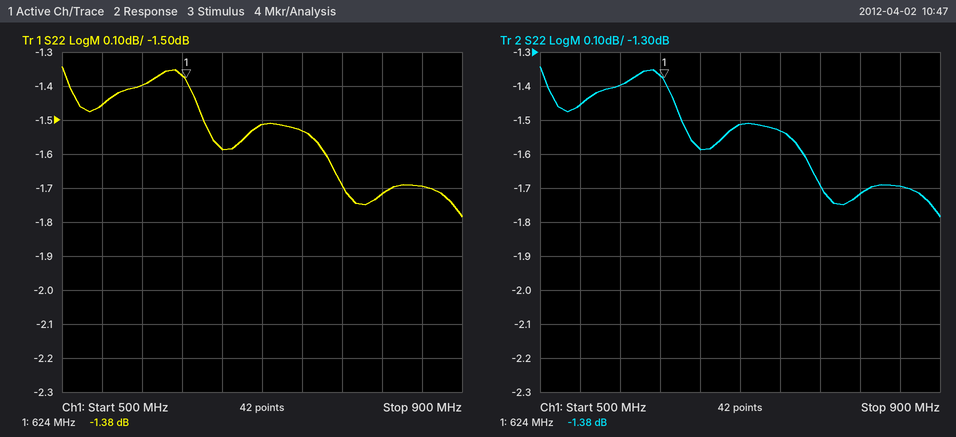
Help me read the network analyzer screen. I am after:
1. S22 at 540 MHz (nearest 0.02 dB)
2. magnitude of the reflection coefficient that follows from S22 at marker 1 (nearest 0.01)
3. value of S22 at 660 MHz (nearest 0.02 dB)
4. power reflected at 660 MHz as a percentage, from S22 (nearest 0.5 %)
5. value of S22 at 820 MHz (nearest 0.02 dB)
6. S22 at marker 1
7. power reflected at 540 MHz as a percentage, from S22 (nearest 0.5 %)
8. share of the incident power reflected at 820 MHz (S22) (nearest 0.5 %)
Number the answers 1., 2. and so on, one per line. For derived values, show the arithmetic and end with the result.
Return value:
1. -1.46 dB
2. 10^(-1.38/20) ≈ 0.85
3. -1.58 dB
4. 10^(-1.58/10) ≈ 69.5 %
5. -1.72 dB
6. -1.38 dB
7. 10^(-1.46/10) ≈ 71.4 %, so 71.5 % to the nearest 0.5 %
8. 10^(-1.72/10) ≈ 67.3 %, so 67.5 % to the nearest 0.5 %
